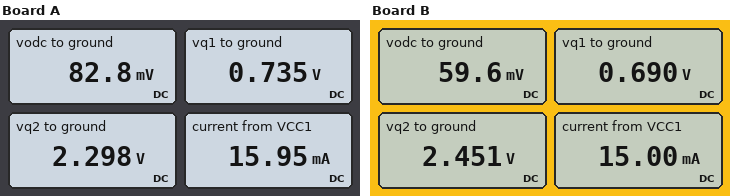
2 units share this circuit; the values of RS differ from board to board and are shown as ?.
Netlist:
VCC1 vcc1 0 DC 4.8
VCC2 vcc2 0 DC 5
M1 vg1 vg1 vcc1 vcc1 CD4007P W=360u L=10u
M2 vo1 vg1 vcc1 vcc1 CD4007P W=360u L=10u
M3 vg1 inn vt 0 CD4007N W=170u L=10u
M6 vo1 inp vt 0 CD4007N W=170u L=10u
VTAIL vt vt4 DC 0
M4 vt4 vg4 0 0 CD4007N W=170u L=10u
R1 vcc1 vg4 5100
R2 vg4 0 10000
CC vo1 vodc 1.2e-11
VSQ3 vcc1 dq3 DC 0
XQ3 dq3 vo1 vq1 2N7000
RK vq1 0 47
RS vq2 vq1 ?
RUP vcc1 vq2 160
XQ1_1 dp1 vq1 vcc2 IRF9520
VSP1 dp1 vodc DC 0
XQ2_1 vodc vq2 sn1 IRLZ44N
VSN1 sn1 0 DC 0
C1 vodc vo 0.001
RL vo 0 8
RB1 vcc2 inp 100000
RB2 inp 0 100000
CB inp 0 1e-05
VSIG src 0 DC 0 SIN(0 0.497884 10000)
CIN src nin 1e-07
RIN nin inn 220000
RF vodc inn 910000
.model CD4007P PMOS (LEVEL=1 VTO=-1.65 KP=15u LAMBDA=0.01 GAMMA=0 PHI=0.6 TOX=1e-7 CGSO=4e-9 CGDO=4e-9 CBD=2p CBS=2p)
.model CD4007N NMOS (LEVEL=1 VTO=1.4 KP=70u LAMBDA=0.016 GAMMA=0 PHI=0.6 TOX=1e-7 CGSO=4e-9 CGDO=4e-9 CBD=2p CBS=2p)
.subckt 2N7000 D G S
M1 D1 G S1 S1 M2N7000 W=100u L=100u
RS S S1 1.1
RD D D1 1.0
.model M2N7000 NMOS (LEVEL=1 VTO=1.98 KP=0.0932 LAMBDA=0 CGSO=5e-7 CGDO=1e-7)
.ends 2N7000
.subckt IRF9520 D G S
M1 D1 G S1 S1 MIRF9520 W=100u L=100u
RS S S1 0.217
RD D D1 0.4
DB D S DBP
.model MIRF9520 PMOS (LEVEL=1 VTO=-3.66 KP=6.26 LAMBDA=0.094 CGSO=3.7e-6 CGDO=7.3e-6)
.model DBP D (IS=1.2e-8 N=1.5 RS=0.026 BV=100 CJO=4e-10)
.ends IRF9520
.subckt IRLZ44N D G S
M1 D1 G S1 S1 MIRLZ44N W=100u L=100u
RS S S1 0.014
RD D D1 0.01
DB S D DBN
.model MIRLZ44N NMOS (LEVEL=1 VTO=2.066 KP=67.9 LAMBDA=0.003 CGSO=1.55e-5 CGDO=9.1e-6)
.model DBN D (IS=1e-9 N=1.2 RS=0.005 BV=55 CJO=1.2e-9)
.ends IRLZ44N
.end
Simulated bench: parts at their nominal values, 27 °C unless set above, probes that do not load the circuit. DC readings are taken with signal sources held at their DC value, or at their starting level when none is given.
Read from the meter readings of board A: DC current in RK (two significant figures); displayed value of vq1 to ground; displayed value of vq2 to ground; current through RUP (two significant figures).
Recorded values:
16 mA
0.735 V
2.298 V
16 mA
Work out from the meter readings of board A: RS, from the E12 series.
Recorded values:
100 Ω
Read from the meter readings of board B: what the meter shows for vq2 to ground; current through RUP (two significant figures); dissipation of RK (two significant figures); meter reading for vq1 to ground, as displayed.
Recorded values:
2.451 V
15 mA
10 mW
0.690 V
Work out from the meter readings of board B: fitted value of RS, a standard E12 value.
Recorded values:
120 Ω
